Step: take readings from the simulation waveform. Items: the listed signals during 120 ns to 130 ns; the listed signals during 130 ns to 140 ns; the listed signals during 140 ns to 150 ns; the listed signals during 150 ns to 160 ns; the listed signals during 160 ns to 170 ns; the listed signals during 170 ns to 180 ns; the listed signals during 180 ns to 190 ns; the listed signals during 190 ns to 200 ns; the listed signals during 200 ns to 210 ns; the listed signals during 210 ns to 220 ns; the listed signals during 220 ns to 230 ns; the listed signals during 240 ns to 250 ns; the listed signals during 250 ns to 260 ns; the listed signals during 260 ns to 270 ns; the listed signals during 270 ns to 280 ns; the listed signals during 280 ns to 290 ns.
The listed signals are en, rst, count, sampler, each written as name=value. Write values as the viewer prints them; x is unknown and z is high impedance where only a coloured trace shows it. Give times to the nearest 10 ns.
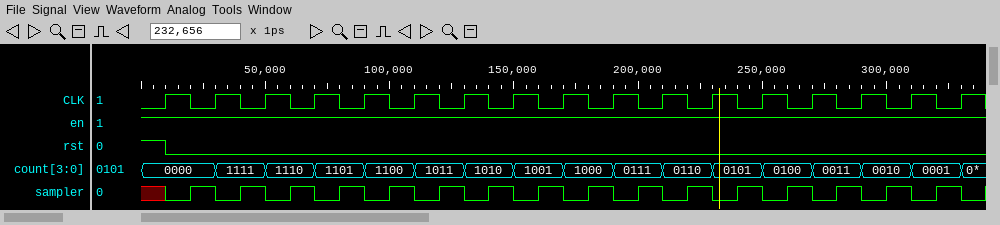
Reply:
en=1, rst=0, count=1011, sampler=1
en=1, rst=0, count=1010, sampler=0
en=1, rst=0, count=1010, sampler=1
en=1, rst=0, count=1001, sampler=0
en=1, rst=0, count=1001, sampler=1
en=1, rst=0, count=1000, sampler=0
en=1, rst=0, count=1000, sampler=1
en=1, rst=0, count=0111, sampler=0
en=1, rst=0, count=0111, sampler=1
en=1, rst=0, count=0110, sampler=0
en=1, rst=0, count=0110, sampler=1
en=1, rst=0, count=0101, sampler=1
en=1, rst=0, count=0100, sampler=0
en=1, rst=0, count=0100, sampler=1
en=1, rst=0, count=0011, sampler=0
en=1, rst=0, count=0011, sampler=1
